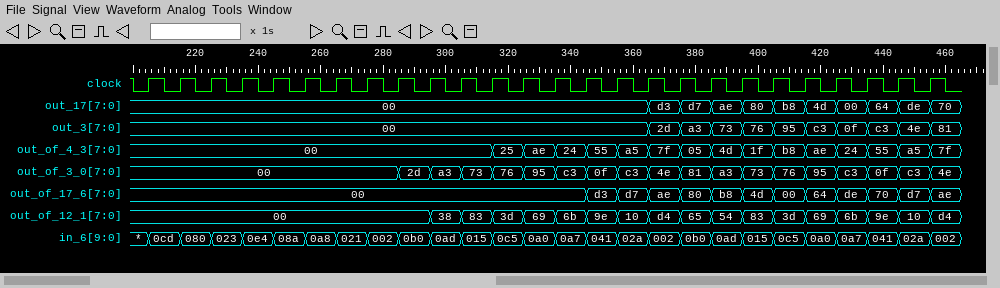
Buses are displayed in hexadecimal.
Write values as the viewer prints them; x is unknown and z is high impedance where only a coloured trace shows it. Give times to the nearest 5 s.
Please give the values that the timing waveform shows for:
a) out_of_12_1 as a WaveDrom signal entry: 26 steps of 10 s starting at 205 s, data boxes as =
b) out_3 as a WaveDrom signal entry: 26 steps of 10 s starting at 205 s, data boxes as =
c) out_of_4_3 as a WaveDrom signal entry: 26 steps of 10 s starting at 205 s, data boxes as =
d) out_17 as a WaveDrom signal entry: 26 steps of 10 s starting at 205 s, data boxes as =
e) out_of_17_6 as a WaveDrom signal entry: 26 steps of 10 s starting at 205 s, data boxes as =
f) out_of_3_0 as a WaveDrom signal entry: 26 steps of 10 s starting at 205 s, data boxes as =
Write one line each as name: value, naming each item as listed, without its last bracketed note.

out_of_12_1 as a WaveDrom signal entry: 26 steps of 10 s starting at 205 s, data boxes as =: {name: 'out_of_12_1', wave: '=........=================', data: '00 38 83 3d 69 6b 9e 10 d4 65 54 83 3d 69 6b 9e 10 d4'}
out_3 as a WaveDrom signal entry: 26 steps of 10 s starting at 205 s, data boxes as =: {name: 'out_3', wave: '=...............==========', data: '00 2d a3 73 76 95 c3 0f c3 4e 81'}
out_of_4_3 as a WaveDrom signal entry: 26 steps of 10 s starting at 205 s, data boxes as =: {name: 'out_of_4_3', wave: '=..........===============', data: '00 25 ae 24 55 a5 7f 05 4d 1f b8 ae 24 55 a5 7f'}
out_17 as a WaveDrom signal entry: 26 steps of 10 s starting at 205 s, data boxes as =: {name: 'out_17', wave: '=...............==========', data: '00 d3 d7 ae 80 b8 4d 00 64 de 70'}
out_of_17_6 as a WaveDrom signal entry: 26 steps of 10 s starting at 205 s, data boxes as =: {name: 'out_of_17_6', wave: '=.............============', data: '00 d3 d7 ae 80 b8 4d 00 64 de 70 d7 ae'}
out_of_3_0 as a WaveDrom signal entry: 26 steps of 10 s starting at 205 s, data boxes as =: {name: 'out_of_3_0', wave: '=.......==================', data: '00 2d a3 73 76 95 c3 0f c3 4e 81 a3 73 76 95 c3 0f c3 4e'}
